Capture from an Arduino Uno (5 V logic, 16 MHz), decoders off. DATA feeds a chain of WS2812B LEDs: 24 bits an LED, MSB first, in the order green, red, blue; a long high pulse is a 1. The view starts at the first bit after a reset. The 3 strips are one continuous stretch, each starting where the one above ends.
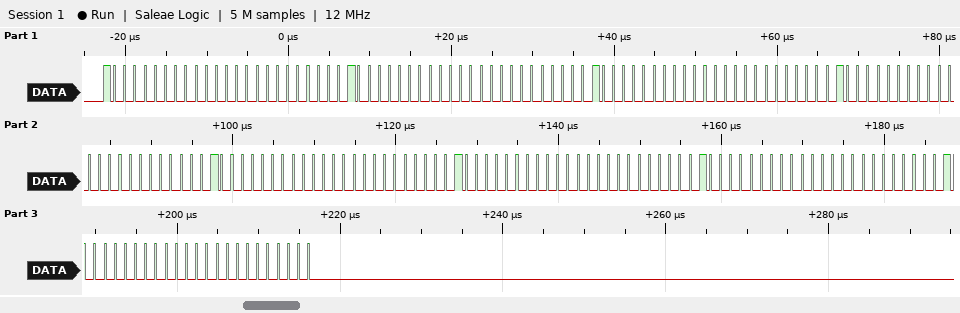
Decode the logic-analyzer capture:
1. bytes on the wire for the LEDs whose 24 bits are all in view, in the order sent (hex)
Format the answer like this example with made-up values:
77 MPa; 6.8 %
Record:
80 00 00 80 00 00 80 00 00 80 00 00 80 00 00 80 00 00 80 00 00 80 00 00
